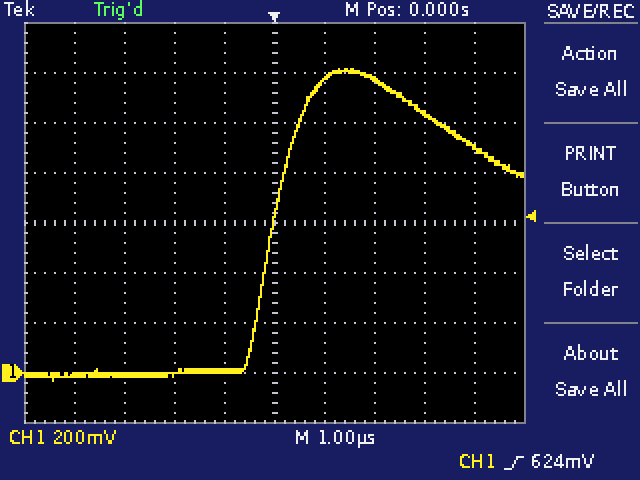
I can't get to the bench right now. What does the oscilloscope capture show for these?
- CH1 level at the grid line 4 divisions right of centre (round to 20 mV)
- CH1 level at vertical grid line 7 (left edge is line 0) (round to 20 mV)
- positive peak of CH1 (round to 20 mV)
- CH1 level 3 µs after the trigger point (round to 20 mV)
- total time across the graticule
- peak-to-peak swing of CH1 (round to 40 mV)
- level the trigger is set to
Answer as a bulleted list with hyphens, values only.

- 900 mV
- 1.18 V
- 1.22 V
- 1.04 V
- 10 µs
- 1.24 V
- 624 mV
